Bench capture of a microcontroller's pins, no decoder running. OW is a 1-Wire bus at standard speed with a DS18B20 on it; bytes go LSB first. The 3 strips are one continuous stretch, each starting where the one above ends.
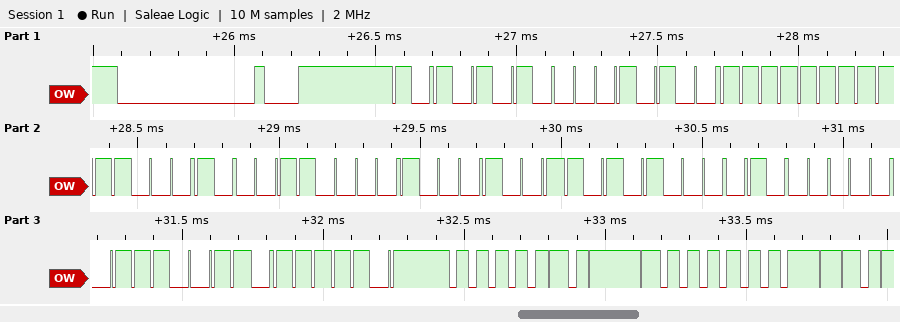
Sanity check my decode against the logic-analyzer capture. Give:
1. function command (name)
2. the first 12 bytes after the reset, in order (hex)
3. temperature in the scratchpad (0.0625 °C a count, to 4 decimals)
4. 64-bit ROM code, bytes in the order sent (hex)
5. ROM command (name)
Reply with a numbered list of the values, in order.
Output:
1. Read Scratchpad
2. 55 28 FF 47 0C 91 15 02 CE BE A0 01
3. 26.0000 °C
4. 28 FF 47 0C 91 15 02 CE
5. Match ROM
